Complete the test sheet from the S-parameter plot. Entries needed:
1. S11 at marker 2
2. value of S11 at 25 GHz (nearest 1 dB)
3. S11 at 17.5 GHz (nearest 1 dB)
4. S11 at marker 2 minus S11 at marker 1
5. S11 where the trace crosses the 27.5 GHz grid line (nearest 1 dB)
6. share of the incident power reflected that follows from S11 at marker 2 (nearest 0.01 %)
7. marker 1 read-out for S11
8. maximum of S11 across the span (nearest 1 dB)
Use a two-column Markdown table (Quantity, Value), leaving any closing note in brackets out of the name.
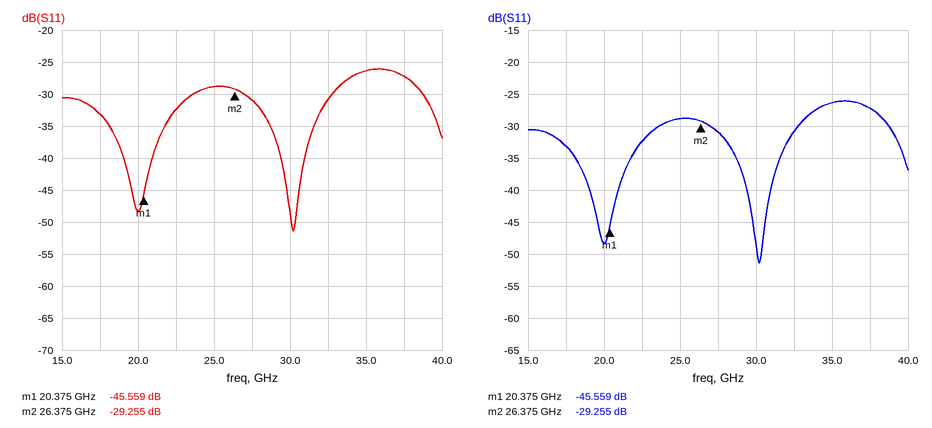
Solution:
| Quantity | Value |
|---|---|
| S11 at marker 2 | -29.255 dB |
| value of S11 at 25 GHz | -29 dB |
| S11 at 17.5 GHz | -33 dB |
| S11 at marker 2 minus S11 at marker 1 | 16.304 dB |
| S11 where the trace crosses the 27.5 GHz grid line | -31 dB |
| share of the incident power reflected that follows from S11 at marker 2 | 0.12 % |
| marker 1 read-out for S11 | -45.559 dB |
| maximum of S11 across the span | -26 dB |
